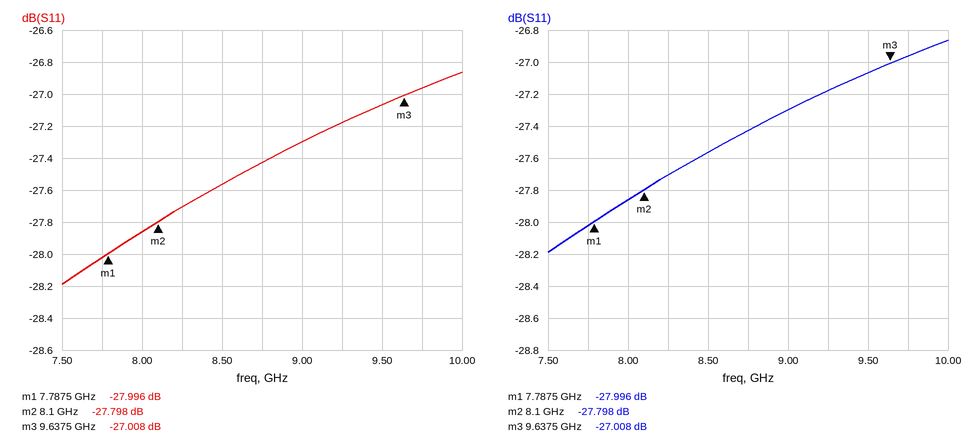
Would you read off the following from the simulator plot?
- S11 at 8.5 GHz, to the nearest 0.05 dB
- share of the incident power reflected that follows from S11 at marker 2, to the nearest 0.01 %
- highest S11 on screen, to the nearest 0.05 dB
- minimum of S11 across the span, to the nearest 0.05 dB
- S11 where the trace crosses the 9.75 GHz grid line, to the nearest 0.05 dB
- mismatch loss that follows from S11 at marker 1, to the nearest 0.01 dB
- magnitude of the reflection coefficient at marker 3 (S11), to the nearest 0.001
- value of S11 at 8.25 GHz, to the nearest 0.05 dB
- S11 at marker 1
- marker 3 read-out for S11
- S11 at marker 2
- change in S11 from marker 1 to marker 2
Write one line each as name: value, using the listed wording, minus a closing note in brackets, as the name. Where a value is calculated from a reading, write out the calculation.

S11 at 8.5 GHz, to the nearest 0.05 dB: -27.55 dB
share of the incident power reflected that follows from S11 at marker 2, to the nearest 0.01 %: 10^(-27.798/10) ≈ 0.17 %
highest S11 on screen, to the nearest 0.05 dB: -26.85 dB
minimum of S11 across the span, to the nearest 0.05 dB: -28.20 dB
S11 where the trace crosses the 9.75 GHz grid line, to the nearest 0.05 dB: -26.95 dB
mismatch loss that follows from S11 at marker 1, to the nearest 0.01 dB: −10 log10(1 − 10^(-27.996/10)) ≈ 0.01 dB
magnitude of the reflection coefficient at marker 3 (S11), to the nearest 0.001: 10^(-27.008/20) ≈ 0.045
value of S11 at 8.25 GHz, to the nearest 0.05 dB: -27.70 dB
S11 at marker 1: -27.996 dB
marker 3 read-out for S11: -27.008 dB
S11 at marker 2: -27.798 dB
change in S11 from marker 1 to marker 2: -27.798 − (-27.996) = 0.198 dB
